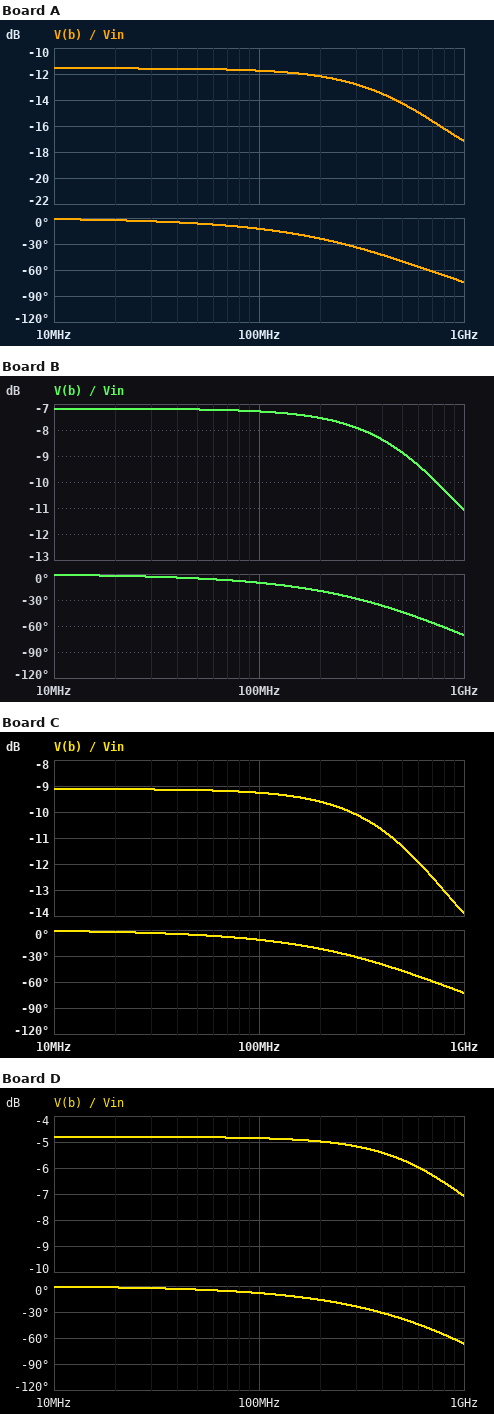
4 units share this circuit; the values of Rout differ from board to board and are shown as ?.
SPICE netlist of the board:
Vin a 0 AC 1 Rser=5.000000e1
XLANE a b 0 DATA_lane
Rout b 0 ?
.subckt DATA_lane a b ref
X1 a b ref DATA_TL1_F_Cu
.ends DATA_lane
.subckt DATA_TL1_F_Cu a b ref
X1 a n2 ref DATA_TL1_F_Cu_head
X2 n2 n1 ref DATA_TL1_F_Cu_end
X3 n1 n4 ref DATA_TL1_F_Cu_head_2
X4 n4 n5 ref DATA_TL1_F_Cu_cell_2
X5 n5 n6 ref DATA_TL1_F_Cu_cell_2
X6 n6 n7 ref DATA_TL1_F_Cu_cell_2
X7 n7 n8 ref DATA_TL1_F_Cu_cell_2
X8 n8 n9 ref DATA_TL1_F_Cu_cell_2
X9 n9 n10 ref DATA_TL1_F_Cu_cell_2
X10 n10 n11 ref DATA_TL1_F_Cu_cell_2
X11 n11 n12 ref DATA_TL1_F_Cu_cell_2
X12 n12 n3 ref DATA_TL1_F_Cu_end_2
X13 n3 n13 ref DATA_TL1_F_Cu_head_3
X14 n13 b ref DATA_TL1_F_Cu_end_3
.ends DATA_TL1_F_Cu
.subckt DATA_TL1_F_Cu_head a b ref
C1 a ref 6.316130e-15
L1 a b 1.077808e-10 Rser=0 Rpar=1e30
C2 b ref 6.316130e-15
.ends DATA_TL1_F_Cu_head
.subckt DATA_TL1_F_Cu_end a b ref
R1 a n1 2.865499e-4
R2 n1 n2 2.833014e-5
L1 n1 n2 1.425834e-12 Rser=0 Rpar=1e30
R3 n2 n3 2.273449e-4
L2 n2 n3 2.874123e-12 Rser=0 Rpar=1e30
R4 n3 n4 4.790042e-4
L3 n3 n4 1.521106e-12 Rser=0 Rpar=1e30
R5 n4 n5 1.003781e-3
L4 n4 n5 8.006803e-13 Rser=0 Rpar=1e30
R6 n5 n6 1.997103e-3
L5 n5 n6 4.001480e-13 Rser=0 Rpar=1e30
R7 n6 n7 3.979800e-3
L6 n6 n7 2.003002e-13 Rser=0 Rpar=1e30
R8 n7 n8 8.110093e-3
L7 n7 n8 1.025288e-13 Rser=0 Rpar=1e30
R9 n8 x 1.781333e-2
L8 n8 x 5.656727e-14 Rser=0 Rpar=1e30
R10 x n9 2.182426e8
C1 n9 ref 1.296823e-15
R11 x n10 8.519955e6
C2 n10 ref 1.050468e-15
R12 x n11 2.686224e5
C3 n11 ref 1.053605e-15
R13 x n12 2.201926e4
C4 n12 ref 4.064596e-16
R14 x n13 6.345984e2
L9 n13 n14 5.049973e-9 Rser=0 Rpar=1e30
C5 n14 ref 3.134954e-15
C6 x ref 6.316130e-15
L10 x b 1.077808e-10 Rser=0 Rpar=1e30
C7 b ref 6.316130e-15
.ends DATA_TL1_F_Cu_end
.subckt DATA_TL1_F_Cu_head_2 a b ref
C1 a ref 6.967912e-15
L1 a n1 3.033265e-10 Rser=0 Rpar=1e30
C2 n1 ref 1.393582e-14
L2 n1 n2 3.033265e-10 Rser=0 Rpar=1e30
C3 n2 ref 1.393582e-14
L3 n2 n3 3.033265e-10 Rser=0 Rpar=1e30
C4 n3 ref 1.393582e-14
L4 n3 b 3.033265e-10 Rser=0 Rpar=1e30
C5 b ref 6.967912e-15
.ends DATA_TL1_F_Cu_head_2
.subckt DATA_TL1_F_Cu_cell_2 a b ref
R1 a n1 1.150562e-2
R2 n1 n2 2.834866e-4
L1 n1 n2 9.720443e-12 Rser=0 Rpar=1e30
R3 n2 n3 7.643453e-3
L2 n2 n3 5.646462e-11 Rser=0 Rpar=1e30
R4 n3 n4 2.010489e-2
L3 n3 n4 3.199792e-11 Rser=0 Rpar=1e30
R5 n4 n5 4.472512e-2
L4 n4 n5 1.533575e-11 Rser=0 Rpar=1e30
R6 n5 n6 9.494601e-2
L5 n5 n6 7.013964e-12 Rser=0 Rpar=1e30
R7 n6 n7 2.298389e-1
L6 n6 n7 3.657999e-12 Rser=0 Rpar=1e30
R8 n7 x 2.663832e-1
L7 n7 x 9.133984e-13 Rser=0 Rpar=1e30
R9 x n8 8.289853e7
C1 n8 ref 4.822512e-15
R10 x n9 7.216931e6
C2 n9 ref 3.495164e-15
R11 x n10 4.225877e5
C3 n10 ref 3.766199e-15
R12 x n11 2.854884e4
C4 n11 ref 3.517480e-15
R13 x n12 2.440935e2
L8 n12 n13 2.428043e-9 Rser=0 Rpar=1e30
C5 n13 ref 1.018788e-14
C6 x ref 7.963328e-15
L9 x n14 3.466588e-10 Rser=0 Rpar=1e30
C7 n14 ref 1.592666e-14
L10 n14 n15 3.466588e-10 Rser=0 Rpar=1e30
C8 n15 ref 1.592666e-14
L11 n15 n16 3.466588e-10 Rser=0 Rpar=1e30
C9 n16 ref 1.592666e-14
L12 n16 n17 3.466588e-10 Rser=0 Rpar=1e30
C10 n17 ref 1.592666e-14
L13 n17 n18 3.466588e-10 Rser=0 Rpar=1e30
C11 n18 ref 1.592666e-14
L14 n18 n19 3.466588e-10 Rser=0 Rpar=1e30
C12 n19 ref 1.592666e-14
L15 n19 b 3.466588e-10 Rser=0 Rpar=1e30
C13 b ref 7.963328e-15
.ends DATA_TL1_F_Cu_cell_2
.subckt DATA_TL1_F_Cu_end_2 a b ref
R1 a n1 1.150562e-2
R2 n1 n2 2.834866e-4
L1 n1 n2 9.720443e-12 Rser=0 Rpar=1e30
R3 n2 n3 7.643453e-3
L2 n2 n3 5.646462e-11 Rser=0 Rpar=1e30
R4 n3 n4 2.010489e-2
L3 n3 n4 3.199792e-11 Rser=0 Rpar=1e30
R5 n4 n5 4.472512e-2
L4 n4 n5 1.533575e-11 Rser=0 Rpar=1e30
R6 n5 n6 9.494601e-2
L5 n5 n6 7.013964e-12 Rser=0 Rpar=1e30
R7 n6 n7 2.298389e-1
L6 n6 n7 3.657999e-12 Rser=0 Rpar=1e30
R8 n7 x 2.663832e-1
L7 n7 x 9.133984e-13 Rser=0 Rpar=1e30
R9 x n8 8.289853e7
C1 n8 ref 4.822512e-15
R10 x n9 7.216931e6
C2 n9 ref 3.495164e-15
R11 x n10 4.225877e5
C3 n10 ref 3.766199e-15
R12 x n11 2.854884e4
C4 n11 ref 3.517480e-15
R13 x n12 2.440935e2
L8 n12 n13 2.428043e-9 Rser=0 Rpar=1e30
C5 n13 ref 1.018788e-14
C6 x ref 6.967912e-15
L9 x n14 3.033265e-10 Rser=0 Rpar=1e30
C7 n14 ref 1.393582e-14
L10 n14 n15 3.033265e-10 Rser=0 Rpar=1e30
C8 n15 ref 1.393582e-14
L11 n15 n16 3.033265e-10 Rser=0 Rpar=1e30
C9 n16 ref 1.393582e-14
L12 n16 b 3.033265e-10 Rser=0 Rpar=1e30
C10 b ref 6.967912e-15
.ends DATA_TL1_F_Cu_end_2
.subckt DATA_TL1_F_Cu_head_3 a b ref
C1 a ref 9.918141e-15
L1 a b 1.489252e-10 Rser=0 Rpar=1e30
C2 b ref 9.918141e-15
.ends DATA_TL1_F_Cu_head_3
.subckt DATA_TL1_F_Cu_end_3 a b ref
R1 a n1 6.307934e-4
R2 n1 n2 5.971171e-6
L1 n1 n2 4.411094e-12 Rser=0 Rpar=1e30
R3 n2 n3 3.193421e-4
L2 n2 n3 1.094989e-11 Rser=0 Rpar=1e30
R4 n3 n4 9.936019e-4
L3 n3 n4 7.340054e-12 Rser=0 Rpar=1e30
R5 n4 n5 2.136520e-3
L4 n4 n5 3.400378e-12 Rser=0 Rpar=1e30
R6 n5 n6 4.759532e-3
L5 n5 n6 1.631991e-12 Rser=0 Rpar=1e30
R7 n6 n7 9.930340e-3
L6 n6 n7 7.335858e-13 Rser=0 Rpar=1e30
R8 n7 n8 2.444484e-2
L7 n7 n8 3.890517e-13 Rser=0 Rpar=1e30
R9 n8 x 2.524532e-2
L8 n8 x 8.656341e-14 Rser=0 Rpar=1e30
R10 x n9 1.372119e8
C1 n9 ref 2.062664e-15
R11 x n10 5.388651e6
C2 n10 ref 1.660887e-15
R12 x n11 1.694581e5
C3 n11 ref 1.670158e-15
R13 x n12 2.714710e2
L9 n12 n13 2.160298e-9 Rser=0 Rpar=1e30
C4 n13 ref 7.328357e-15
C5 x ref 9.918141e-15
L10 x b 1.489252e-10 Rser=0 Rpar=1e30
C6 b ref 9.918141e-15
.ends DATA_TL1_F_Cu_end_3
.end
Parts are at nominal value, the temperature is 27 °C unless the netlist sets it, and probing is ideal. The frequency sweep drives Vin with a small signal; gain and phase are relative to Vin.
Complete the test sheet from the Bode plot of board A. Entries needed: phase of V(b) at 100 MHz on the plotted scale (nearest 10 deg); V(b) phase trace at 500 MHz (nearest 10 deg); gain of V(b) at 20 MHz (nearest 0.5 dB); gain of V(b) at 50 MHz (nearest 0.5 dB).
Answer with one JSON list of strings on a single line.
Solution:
["-10 deg", "-50 deg", "-11.5 dB", "-11.5 dB"]
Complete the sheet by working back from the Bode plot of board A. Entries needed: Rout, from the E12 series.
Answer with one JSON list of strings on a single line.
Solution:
["18 Ω"]
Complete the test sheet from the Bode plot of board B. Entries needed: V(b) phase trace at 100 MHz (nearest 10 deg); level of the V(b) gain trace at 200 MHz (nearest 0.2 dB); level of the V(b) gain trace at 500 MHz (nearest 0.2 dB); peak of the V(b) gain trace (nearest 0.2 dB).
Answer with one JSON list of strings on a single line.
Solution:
["-10 deg", "-7.6 dB", "-8.8 dB", "-7.2 dB"]
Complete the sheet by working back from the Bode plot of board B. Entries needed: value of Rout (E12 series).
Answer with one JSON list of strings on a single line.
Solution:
["39 Ω"]
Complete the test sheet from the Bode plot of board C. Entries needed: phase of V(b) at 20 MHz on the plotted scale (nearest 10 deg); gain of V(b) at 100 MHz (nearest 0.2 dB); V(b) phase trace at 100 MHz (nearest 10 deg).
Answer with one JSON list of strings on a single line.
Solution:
["0 deg", "-9.2 dB", "-10 deg"]
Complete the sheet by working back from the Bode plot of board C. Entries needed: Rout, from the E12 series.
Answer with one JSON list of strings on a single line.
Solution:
["27 Ω"]
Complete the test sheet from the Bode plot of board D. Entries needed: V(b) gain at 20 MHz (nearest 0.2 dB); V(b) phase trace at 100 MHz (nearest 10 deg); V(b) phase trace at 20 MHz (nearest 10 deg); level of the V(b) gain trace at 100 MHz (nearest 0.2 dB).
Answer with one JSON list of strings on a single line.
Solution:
["-4.8 dB", "-10 deg", "0 deg", "-4.8 dB"]
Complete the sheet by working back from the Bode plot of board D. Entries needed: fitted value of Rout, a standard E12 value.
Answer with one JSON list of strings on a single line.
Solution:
["68 Ω"]
